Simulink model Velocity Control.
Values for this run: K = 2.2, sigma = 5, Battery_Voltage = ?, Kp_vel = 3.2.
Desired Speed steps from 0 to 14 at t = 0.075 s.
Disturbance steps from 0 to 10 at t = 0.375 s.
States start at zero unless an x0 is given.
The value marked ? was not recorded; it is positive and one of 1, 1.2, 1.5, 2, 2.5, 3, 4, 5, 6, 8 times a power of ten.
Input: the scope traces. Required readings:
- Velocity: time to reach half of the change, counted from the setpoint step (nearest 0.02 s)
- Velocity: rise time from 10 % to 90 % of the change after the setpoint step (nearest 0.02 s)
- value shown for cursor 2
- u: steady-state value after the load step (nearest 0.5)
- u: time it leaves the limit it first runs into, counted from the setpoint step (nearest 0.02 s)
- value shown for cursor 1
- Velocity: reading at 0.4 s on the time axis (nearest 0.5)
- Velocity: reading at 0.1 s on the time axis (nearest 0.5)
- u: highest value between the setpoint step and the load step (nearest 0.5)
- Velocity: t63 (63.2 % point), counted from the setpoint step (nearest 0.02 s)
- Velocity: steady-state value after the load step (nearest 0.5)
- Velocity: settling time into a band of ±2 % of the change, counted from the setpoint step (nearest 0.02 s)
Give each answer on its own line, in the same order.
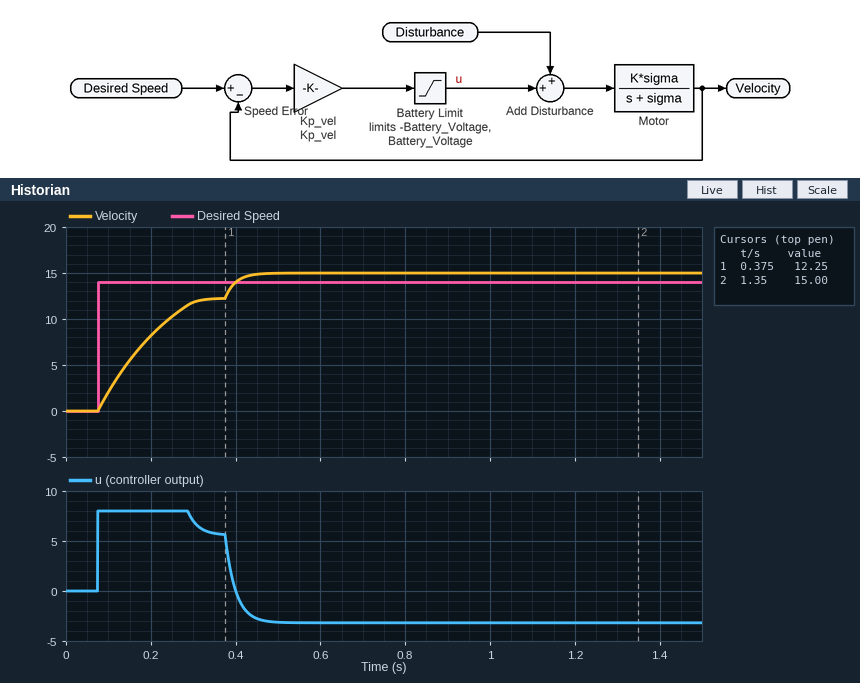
0.08 s
0.18 s
15.00
-3.0
0.22 s
12.25
14.0
2.0
8.0
0.12 s
15.0
0.24 s
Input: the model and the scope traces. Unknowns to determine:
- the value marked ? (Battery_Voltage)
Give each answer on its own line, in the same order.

8
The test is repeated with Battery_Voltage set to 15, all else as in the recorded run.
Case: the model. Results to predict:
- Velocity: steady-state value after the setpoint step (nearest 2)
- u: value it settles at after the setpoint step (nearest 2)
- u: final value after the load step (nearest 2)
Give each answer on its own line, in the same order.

12
6
-4
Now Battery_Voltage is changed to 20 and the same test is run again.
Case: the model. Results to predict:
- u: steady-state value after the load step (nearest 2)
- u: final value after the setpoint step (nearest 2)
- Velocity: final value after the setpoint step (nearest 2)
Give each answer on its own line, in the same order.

-4
6
12
